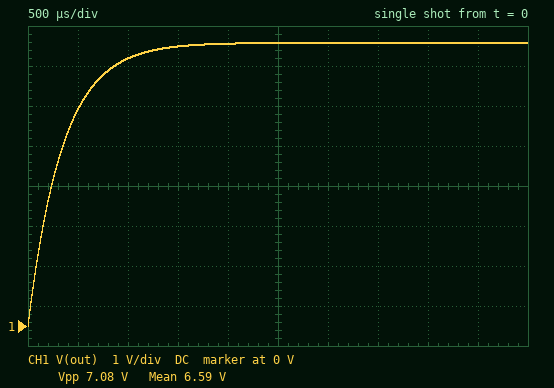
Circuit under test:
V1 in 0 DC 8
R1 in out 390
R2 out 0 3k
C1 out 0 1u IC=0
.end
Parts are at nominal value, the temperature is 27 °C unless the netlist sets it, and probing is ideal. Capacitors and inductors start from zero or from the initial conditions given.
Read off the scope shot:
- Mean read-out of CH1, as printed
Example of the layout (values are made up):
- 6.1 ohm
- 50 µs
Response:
- 6.59 V
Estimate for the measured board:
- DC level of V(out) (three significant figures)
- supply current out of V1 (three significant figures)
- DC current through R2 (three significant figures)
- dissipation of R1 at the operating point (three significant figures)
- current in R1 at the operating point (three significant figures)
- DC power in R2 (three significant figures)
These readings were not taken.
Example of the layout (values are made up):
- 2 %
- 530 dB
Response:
- 7.08 V
- 2.36 mA
- 2.36 mA
- 2.17 mW
- 2.36 mA
- 16.7 mW
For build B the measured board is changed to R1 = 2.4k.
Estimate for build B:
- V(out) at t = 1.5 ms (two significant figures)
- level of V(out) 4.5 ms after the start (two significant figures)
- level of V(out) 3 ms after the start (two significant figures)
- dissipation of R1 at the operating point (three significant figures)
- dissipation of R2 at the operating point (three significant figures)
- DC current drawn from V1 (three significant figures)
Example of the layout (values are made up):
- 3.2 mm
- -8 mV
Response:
- 3.0 V
- 4.3 V
- 4.0 V
- 5.27 mW
- 6.58 mW
- 1.48 mA
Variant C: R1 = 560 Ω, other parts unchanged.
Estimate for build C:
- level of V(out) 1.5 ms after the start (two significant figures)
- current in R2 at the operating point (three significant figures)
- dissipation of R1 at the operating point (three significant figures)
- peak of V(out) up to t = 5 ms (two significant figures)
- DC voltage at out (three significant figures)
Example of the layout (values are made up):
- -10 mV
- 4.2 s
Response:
- 6.5 V
- 2.25 mA
- 2.83 mW
- 6.7 V
- 6.74 V
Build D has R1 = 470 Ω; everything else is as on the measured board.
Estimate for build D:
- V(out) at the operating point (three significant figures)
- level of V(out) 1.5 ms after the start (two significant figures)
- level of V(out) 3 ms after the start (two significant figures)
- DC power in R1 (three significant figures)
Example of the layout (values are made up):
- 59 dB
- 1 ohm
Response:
- 6.92 V
- 6.7 V
- 6.9 V
- 2.50 mW
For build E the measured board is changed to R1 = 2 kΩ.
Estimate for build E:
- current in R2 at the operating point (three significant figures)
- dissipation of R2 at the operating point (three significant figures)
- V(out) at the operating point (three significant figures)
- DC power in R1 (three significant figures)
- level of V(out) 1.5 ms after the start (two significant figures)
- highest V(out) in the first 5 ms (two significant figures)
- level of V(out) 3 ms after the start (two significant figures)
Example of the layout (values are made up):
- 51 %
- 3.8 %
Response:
- 1.60 mA
- 7.68 mW
- 4.80 V
- 5.12 mW
- 3.4 V
- 4.7 V
- 4.4 V
